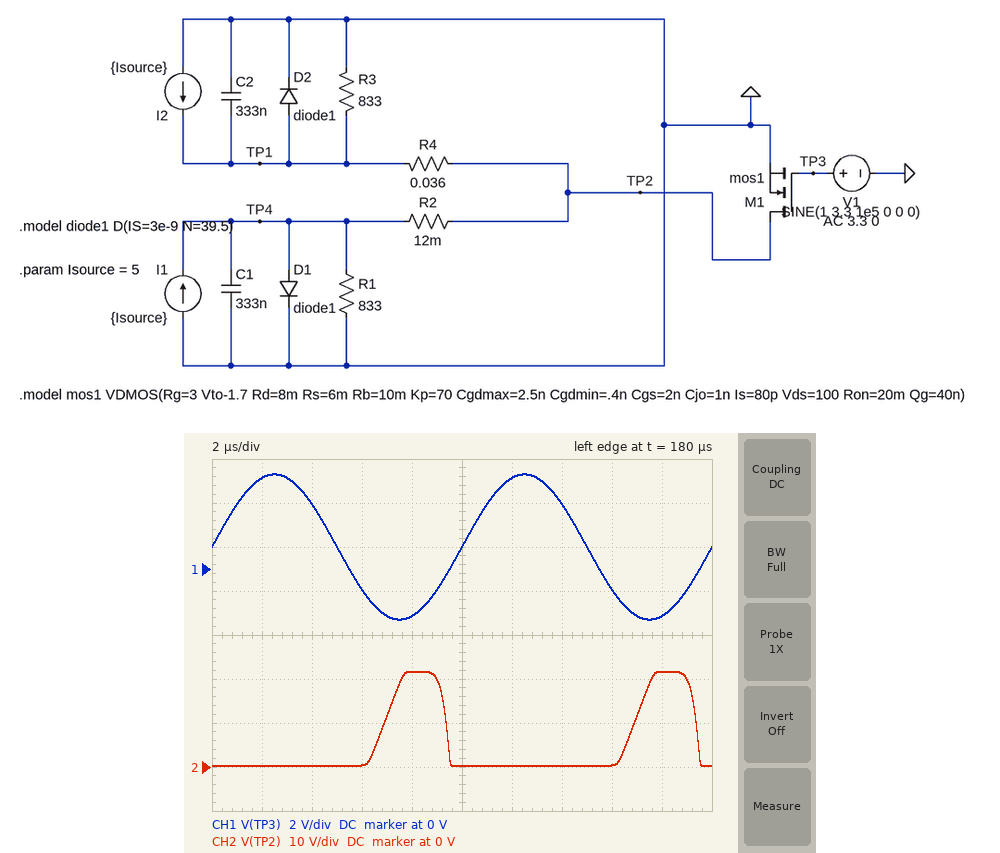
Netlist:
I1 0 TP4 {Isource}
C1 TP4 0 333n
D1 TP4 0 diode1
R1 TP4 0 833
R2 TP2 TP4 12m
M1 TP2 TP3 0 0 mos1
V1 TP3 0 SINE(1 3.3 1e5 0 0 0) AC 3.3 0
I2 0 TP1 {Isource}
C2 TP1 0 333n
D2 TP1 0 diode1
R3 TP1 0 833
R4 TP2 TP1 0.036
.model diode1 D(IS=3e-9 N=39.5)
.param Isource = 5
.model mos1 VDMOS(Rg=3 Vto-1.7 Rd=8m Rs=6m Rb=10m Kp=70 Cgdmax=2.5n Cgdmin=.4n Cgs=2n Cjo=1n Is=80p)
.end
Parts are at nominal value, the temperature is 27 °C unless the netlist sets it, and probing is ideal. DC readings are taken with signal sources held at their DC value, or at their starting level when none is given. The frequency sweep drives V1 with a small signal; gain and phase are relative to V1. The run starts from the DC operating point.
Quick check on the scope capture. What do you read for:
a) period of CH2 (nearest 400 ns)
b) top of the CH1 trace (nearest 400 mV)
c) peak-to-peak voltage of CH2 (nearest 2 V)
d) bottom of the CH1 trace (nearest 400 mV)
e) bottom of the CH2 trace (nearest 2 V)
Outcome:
10.0 µs
4.4 V
22 V
-2.4 V
0 V
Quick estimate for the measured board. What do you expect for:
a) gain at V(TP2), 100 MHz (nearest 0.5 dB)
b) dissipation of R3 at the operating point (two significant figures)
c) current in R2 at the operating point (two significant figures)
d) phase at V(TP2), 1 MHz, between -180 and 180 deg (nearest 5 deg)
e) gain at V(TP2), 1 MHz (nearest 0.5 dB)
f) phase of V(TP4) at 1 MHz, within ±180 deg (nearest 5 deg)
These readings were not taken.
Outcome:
-57.5 dB
170 µW
5.0 A
170 deg
-33.5 dB
170 deg
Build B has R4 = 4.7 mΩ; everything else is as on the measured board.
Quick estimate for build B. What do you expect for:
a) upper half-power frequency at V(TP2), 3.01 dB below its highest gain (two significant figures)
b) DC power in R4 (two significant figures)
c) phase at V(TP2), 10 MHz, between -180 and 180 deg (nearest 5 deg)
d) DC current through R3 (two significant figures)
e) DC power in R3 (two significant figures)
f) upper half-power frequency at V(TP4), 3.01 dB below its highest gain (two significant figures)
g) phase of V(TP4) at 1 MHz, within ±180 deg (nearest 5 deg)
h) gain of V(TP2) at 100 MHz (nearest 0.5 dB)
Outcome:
7.2 MHz
120 mW
100 deg
260 µA
57 µW
7.0 MHz
170 deg
-62.5 dB
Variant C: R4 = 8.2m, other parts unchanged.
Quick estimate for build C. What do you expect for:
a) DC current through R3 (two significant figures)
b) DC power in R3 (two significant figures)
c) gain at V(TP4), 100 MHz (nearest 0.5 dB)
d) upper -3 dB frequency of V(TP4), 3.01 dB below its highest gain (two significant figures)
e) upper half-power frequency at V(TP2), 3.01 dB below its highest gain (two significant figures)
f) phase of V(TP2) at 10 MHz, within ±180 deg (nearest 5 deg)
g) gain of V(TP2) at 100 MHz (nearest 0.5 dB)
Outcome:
280 µA
67 µW
-70.0 dB
6.9 MHz
7.1 MHz
100 deg
-61.0 dB
